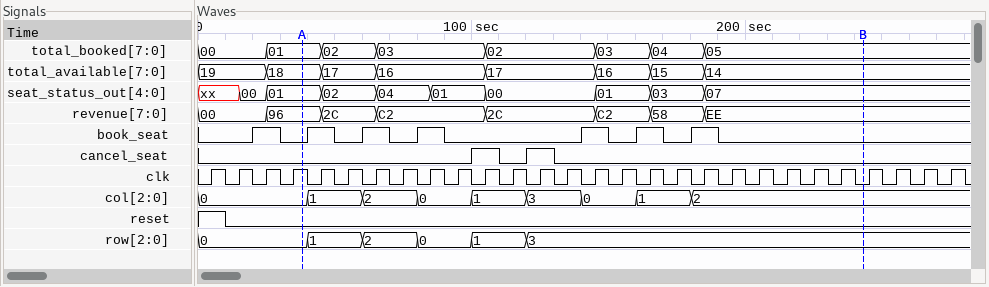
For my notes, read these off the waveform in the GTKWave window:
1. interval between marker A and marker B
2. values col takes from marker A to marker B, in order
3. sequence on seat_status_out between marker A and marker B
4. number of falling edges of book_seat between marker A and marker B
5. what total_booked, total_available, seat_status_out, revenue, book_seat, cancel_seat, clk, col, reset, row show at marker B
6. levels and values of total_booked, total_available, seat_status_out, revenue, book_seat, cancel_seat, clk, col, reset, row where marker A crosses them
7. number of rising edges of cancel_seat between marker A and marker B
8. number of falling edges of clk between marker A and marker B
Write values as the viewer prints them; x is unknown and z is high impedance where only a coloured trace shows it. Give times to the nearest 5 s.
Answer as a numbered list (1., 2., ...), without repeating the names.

1. 205 s
2. 0, 1, 2, 0, 1, 3, 0, 1, 2
3. 01, 02, 04, 01, 00, 01, 03, 07
4. 6
5. total_booked=05, total_available=14, seat_status_out=07, revenue=EE, book_seat=0, cancel_seat=0, clk=0, col=2, reset=0, row=3
6. total_booked=01, total_available=18, seat_status_out=01, revenue=96, book_seat=0, cancel_seat=0, clk=1, col=0, reset=0, row=0
7. 2
8. 21
